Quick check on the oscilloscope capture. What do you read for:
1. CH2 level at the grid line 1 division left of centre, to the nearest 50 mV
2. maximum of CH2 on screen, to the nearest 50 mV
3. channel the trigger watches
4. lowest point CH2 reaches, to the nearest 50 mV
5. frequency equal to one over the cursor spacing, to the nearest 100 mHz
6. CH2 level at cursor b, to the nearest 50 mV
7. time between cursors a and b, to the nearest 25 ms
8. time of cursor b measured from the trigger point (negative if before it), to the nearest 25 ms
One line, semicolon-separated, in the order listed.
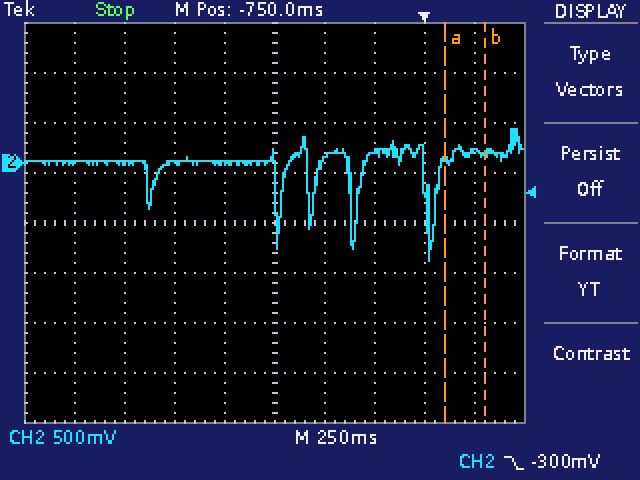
0 mV; 350 mV; CH2; -1.00 V; 5.0 Hz; 100 mV; 200 ms; +300 ms
